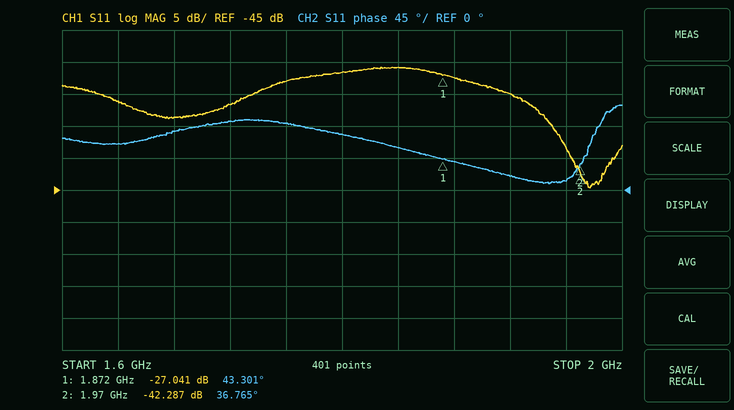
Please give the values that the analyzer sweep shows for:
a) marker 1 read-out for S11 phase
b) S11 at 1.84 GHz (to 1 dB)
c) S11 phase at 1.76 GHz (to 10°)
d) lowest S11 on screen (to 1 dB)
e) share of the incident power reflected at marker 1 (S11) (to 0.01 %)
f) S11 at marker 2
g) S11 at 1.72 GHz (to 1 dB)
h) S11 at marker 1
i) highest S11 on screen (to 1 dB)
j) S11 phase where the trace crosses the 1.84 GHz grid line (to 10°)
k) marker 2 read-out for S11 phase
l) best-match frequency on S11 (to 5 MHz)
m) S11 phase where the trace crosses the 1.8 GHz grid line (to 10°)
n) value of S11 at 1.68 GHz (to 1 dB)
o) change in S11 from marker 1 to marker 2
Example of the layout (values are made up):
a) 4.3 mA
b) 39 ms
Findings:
a) 43.301°
b) -26 dB
c) 90°
d) -45 dB
e) 0.20 %
f) -42.287 dB
g) -32 dB
h) -27.041 dB
i) -26 dB
j) 60°
k) 36.765°
l) 1.975 GHz
m) 80°
n) -34 dB
o) -15.246 dB
